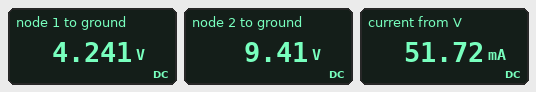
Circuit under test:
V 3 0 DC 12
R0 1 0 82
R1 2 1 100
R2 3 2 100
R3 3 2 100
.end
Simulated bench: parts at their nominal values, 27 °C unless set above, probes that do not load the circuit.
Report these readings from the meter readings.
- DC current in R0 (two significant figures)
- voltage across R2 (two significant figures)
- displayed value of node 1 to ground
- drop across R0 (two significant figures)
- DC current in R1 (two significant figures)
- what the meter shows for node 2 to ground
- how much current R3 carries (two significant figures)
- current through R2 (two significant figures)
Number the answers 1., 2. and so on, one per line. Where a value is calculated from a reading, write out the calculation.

1. (4.241 V) / 82 Ω = 52 mA
2. 12 V - 9.41 V = 2.6 V
3. 4.241 V
4. 4.241 V = 4.2 V
5. (9.41 V - 4.241 V) / 100 Ω = 52 mA
6. 9.41 V
7. (12 V - 9.41 V) / 100 Ω = 26 mA
8. (12 V - 9.41 V) / 100 Ω = 26 mA
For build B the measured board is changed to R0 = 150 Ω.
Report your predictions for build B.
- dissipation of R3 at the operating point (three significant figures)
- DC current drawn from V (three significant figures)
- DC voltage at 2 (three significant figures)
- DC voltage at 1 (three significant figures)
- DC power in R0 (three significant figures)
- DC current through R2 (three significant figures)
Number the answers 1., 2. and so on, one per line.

1. 40.0 mW
2. 40.0 mA
3. 10.0 V
4. 6.00 V
5. 240 mW
6. 20.0 mA
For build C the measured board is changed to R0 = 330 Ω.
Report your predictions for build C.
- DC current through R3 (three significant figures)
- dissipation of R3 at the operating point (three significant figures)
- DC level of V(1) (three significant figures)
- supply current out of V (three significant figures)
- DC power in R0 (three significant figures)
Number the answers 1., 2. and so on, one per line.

1. 12.5 mA
2. 15.6 mW
3. 8.25 V
4. 25.0 mA
5. 206 mW
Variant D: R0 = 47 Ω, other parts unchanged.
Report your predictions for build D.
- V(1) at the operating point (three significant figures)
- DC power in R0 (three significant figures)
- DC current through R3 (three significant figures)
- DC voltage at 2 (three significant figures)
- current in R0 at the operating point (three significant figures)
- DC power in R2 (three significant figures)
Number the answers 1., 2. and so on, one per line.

1. 2.86 V
2. 174 mW
3. 30.5 mA
4. 8.95 V
5. 60.9 mA
6. 92.8 mW
